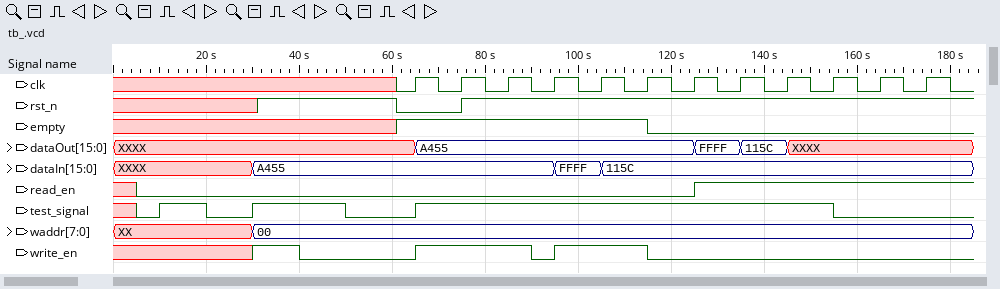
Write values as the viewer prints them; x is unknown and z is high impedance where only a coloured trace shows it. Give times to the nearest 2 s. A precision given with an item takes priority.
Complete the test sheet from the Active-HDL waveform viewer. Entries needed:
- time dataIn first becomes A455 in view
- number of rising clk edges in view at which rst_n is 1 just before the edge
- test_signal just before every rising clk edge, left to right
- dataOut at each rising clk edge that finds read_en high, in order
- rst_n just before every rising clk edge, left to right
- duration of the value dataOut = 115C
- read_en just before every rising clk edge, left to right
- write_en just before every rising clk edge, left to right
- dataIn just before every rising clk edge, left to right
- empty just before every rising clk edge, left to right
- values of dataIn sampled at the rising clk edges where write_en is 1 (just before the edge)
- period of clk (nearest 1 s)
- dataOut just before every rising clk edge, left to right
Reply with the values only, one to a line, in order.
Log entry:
30 s
10
0 1 1 1 1 1 1 1 1 1 0 0
FFFF, 115C, XXXX, XXXX, XXXX
0 0 1 1 1 1 1 1 1 1 1 1
10 s
0 0 0 0 0 0 0 1 1 1 1 1
0 1 1 0 1 1 0 0 0 0 0 0
A455, A455, A455, A455, FFFF, 115C, 115C, 115C, 115C, 115C, 115C, 115C
1 1 1 1 1 1 0 0 0 0 0 0
A455, A455, FFFF, 115C
10 s
XXXX, A455, A455, A455, A455, A455, A455, FFFF, 115C, XXXX, XXXX, XXXX
